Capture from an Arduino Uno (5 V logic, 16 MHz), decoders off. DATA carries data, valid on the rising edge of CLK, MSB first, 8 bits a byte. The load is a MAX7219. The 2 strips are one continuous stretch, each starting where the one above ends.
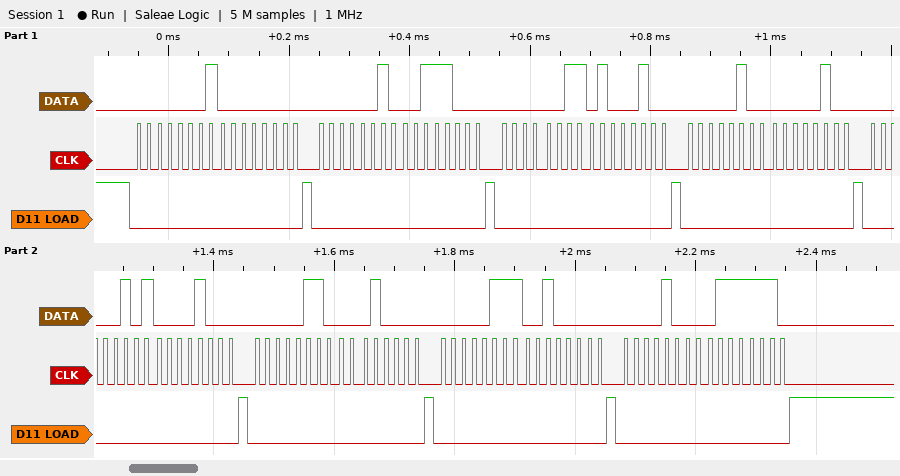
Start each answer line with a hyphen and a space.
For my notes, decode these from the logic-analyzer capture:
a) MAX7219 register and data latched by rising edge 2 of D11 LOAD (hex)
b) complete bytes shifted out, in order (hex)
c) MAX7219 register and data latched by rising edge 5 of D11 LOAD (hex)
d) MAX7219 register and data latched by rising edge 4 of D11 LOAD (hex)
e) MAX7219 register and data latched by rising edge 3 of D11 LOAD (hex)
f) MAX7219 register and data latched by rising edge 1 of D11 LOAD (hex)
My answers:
- register 0x2, data 0x38
- 01 00 02 38 03 44 04 04 05 08 06 10 07 20 08 7E
- register 0x5, data 0x08
- register 0x4, data 0x04
- register 0x3, data 0x44
- register 0x1, data 0x00
